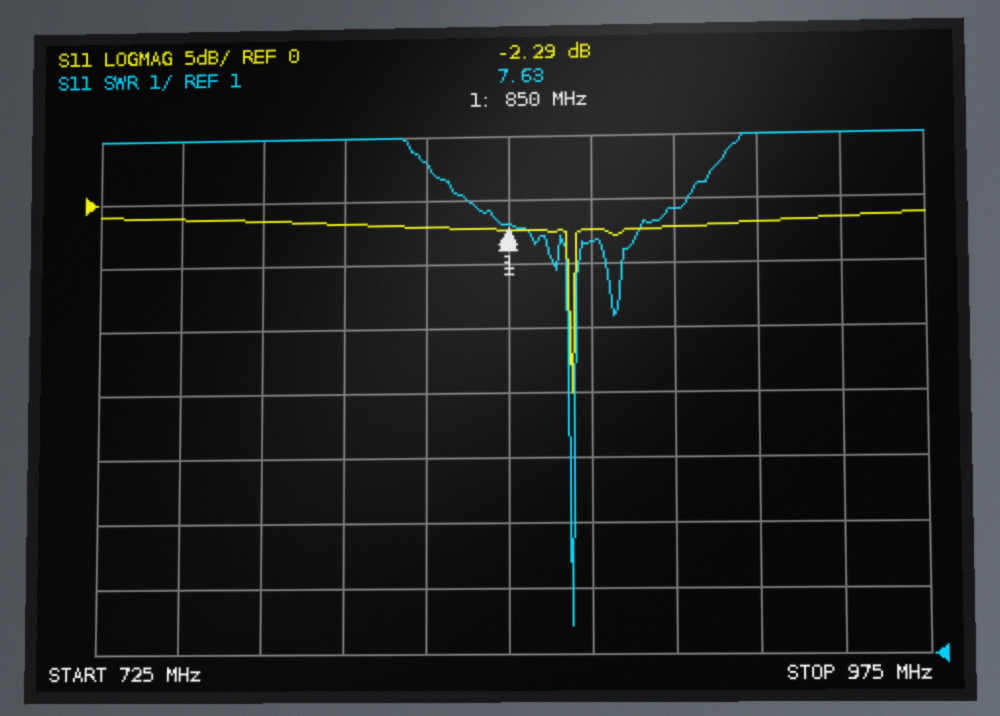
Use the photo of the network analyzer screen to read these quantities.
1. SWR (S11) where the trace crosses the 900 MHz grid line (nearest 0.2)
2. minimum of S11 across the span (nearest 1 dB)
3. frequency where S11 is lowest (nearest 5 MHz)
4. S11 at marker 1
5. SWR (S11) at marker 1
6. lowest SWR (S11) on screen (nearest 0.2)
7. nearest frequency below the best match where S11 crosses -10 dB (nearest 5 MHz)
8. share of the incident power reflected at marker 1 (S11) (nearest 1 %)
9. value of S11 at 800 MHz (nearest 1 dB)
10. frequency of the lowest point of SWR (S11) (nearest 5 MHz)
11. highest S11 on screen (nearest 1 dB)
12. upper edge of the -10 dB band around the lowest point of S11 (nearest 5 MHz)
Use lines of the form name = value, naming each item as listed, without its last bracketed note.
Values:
SWR (S11) where the trace crosses the 900 MHz grid line = 7.8
minimum of S11 across the span = -15 dB
frequency where S11 is lowest = 870 MHz
S11 at marker 1 = -2.29 dB
SWR (S11) at marker 1 = 7.63
lowest SWR (S11) on screen = 1.4
nearest frequency below the best match where S11 crosses -10 dB = 870 MHz
share of the incident power reflected at marker 1 (S11) = 59 %
value of S11 at 800 MHz = -2 dB
frequency of the lowest point of SWR (S11) = 870 MHz
highest S11 on screen = -1 dB
upper edge of the -10 dB band around the lowest point of S11 = 870 MHz
